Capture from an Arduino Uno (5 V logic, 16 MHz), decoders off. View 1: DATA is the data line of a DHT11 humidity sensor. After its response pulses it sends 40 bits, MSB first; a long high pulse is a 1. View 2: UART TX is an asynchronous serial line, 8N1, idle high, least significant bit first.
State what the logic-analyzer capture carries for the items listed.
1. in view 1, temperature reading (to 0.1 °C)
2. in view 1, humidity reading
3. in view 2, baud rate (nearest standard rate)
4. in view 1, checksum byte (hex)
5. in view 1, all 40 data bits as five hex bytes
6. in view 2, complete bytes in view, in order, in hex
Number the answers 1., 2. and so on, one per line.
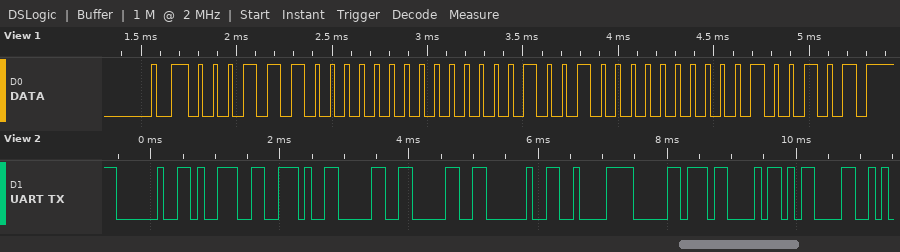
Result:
1. 9.0 °C
2. 28 %
3. 9600 baud
4. 0x25
5. 1C 00 09 00 25
6. 20 39 2E 30 30 20 C2 B0 43 0D
